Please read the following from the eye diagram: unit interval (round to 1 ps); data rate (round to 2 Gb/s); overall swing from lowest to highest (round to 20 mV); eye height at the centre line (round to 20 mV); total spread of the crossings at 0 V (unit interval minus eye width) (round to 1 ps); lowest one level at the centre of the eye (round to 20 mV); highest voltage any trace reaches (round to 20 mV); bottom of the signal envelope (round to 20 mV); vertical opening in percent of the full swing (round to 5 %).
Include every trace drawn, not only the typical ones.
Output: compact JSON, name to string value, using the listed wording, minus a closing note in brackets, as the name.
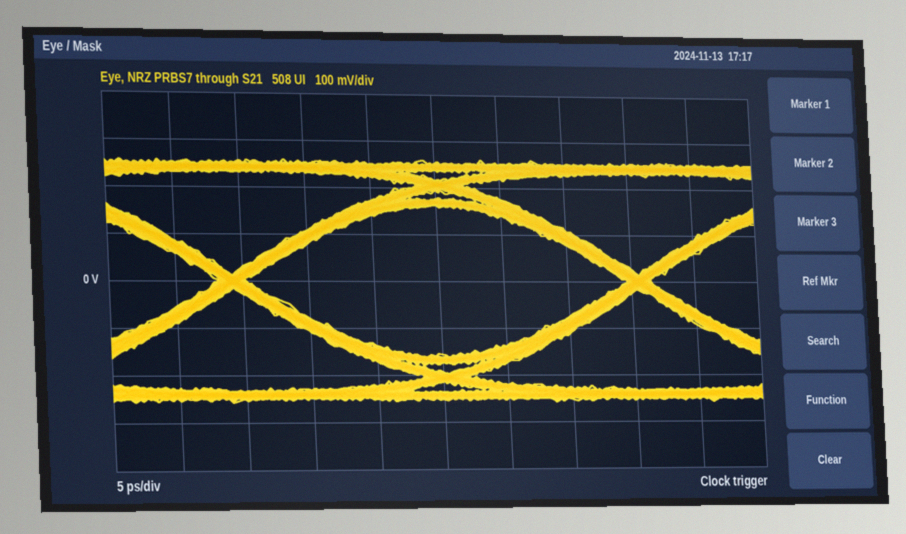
{"unit interval": "31 ps", "data rate": "32 Gb/s", "overall swing from lowest to highest": "520 mV", "eye height at the centre line": "320 mV", "total spread of the crossings at 0 V (unit interval minus eye width)": "2 ps", "lowest one level at the centre of the eye": "160 mV", "highest voltage any trace reaches": "260 mV", "bottom of the signal envelope": "-260 mV", "vertical opening in percent of the full swing": "60 %"}
